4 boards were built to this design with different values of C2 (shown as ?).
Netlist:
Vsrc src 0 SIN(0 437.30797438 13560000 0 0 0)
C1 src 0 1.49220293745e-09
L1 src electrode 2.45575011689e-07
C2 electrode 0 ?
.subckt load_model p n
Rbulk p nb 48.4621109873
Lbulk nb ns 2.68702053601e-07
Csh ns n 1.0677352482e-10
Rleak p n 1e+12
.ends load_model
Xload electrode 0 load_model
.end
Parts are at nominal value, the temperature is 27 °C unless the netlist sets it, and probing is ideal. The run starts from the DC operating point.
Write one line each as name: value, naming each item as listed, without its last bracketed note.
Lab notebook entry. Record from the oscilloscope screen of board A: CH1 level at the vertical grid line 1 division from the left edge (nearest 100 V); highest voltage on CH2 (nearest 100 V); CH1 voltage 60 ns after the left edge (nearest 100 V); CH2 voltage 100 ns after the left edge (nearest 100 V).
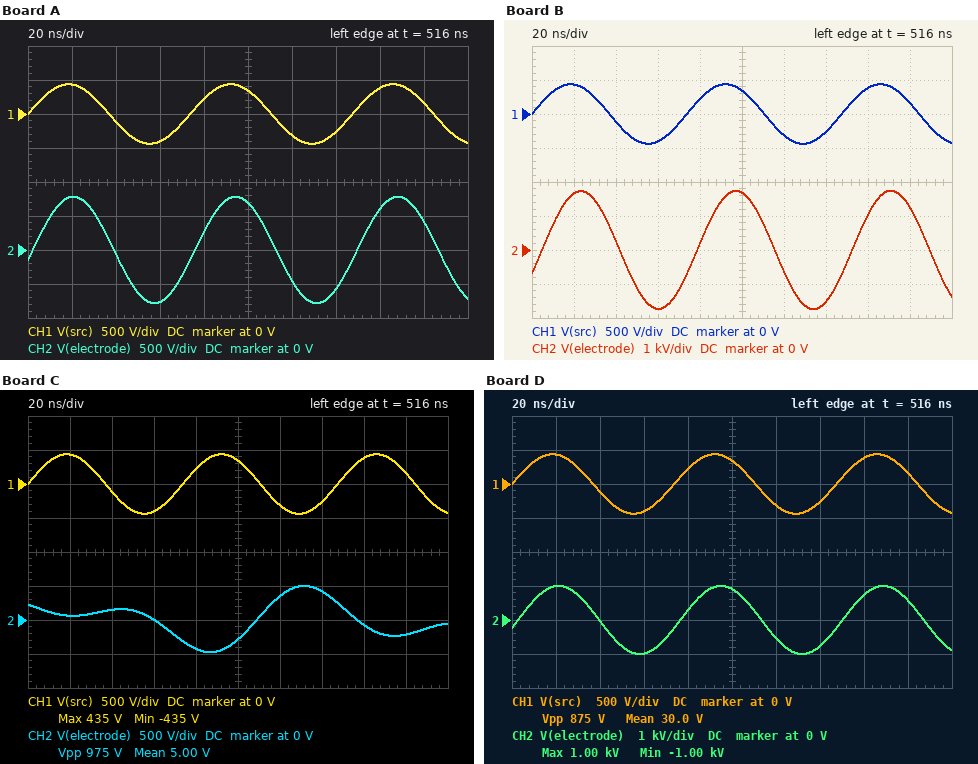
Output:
CH1 level at the vertical grid line 1 division from the left edge: 400 V
highest voltage on CH2: 800 V
CH1 voltage 60 ns after the left edge: -400 V
CH2 voltage 100 ns after the left edge: 700 V
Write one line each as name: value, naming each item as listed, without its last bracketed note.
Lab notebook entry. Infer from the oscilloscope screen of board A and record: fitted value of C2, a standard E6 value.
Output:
fitted value of C2, a standard E6 value: 150 pF
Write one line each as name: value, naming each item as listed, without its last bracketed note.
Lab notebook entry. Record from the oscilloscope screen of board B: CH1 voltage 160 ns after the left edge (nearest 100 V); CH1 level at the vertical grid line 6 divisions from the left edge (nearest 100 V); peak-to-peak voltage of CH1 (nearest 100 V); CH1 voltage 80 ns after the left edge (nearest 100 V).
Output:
CH1 voltage 160 ns after the left edge: 400 V
CH1 level at the vertical grid line 6 divisions from the left edge: -300 V
peak-to-peak voltage of CH1: 900 V
CH1 voltage 80 ns after the left edge: 200 V
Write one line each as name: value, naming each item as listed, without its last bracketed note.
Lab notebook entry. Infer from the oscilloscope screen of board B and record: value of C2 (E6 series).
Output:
value of C2: 330 pF
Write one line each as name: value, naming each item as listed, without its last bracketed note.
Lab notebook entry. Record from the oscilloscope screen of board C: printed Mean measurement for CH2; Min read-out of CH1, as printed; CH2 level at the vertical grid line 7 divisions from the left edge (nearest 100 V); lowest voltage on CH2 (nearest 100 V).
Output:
printed Mean measurement for CH2: 5.00 V
Min read-out of CH1, as printed: -435 V
CH2 level at the vertical grid line 7 divisions from the left edge: 400 V
lowest voltage on CH2: -500 V
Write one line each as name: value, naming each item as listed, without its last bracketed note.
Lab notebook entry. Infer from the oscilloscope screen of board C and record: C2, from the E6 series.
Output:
C2, from the E6 series: 1.5 nF
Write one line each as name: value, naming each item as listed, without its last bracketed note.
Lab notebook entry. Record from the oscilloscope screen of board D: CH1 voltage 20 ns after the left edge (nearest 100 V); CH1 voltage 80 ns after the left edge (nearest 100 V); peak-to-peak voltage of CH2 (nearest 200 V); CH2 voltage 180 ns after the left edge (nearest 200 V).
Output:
CH1 voltage 20 ns after the left edge: 400 V
CH1 voltage 80 ns after the left edge: 200 V
peak-to-peak voltage of CH2: 2.0 kV
CH2 voltage 180 ns after the left edge: 600 V
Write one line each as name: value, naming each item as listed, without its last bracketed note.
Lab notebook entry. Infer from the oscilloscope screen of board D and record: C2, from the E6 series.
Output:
C2, from the E6 series: 220 pF
